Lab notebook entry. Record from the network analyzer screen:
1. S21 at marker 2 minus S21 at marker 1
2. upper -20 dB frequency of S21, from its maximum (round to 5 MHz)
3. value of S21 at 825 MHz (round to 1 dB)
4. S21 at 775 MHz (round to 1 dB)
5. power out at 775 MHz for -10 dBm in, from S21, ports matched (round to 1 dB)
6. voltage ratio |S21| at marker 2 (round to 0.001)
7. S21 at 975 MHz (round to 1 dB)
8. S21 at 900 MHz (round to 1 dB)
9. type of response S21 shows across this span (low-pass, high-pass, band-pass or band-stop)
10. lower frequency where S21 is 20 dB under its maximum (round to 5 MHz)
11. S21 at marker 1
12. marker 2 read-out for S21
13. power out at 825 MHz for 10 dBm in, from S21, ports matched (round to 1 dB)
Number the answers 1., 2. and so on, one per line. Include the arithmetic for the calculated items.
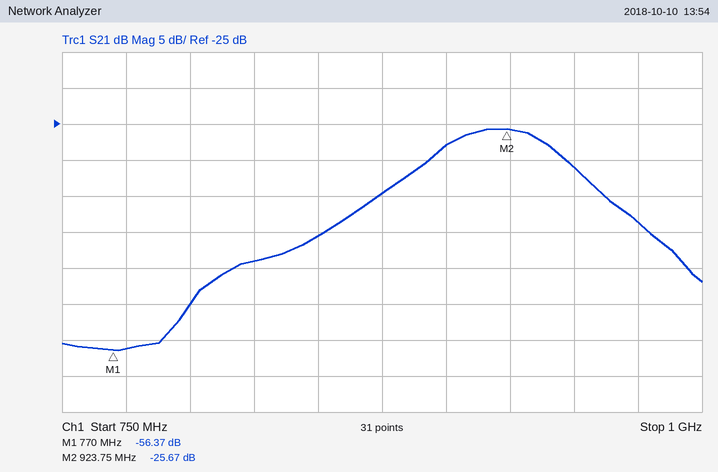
1. -25.67 − (-56.37) = 30.70 dB
2. 995 MHz
3. -44 dB
4. -56 dB
5. -10 dBm + (-56 dB) = -66 dBm
6. 10^(-25.67/20) ≈ 0.052
7. -39 dB
8. -28 dB
9. band-pass
10. 815 MHz
11. -56.37 dB
12. -25.67 dB
13. 10 dBm + (-44 dB) = -34 dBm
